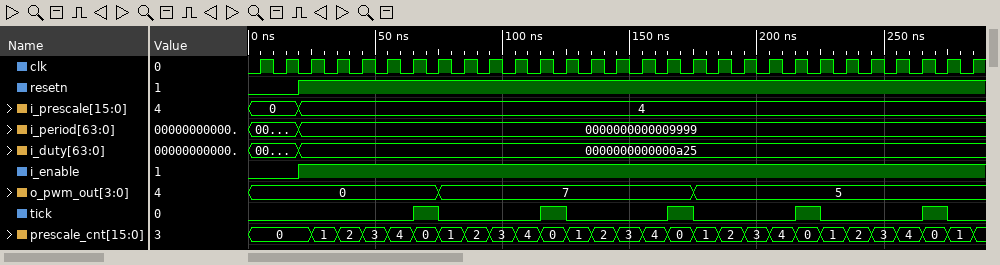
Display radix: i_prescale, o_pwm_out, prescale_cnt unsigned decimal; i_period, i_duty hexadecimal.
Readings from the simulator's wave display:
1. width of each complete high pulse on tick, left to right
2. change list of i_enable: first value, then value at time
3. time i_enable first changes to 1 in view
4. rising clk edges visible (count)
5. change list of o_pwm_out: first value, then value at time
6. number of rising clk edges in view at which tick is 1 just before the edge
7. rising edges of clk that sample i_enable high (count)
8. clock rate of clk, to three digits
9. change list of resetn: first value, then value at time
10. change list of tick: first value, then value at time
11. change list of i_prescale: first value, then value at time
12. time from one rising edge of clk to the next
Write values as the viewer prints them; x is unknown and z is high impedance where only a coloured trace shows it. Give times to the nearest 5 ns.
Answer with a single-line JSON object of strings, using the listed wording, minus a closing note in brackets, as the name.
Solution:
{"width of each complete high pulse on tick, left to right": "10 ns, 10 ns, 10 ns, 10 ns, 10 ns", "change list of i_enable: first value, then value at time": "0, 1 at 20 ns", "time i_enable first changes to 1 in view": "20 ns", "rising clk edges visible": "29", "change list of o_pwm_out: first value, then value at time": "0, 7 at 75 ns, 5 at 175 ns", "number of rising clk edges in view at which tick is 1 just before the edge": "5", "rising edges of clk that sample i_enable high": "27", "clock rate of clk, to three digits": "100 MHz", "change list of resetn: first value, then value at time": "0, 1 at 20 ns", "change list of tick: first value, then value at time": "0, 1 at 65 ns, 0 at 75 ns, 1 at 115 ns, 0 at 125 ns, 1 at 165 ns, 0 at 175 ns, 1 at 215 ns, 0 at 225 ns, 1 at 265 ns, 0 at 275 ns", "change list of i_prescale: first value, then value at time": "0, 4 at 20 ns", "time from one rising edge of clk to the next": "10 ns"}
